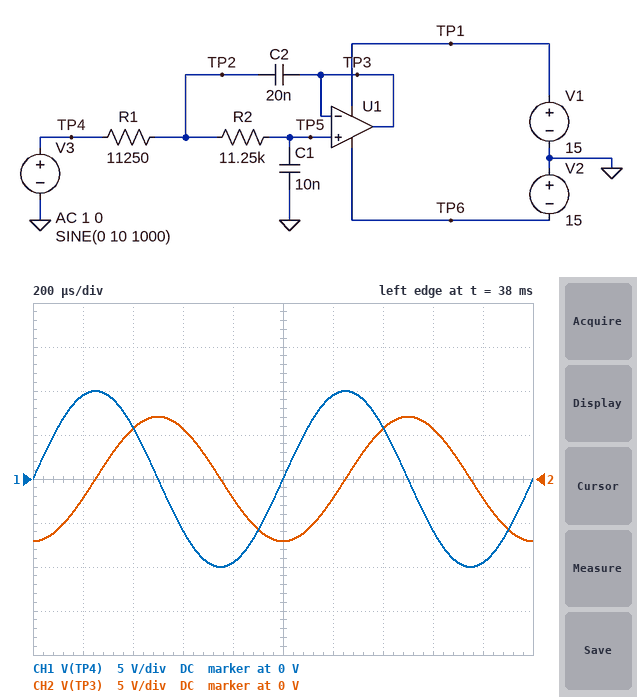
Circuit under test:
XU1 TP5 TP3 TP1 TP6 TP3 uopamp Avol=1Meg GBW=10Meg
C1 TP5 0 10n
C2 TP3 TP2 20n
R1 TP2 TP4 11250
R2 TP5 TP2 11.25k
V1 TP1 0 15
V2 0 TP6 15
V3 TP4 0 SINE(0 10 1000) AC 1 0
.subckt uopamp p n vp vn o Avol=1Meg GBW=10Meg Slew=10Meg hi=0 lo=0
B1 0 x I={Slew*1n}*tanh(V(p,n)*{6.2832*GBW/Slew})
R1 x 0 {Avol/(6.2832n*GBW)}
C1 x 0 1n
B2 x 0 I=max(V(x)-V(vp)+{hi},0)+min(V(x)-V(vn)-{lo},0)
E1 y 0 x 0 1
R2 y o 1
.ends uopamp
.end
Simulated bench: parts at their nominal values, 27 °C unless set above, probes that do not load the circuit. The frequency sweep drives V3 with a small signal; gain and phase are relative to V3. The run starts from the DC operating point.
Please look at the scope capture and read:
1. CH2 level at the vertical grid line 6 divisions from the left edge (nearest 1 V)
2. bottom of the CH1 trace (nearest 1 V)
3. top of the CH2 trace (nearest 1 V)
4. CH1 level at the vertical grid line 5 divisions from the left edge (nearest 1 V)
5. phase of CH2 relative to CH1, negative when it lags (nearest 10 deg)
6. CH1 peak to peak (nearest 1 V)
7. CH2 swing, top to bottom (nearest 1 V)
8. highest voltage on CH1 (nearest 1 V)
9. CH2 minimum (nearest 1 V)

-2 V
-10 V
7 V
0 V
-90 deg
20 V
14 V
10 V
-7 V
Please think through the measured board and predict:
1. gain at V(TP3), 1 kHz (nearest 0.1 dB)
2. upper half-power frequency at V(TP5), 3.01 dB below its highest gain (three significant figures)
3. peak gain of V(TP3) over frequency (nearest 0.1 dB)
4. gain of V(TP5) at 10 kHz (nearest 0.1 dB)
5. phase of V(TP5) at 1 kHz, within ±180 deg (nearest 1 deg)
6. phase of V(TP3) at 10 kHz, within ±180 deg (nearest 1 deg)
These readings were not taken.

-3.0 dB
1.00 kHz
0 dB
-40.0 dB
-90 deg
-172 deg
